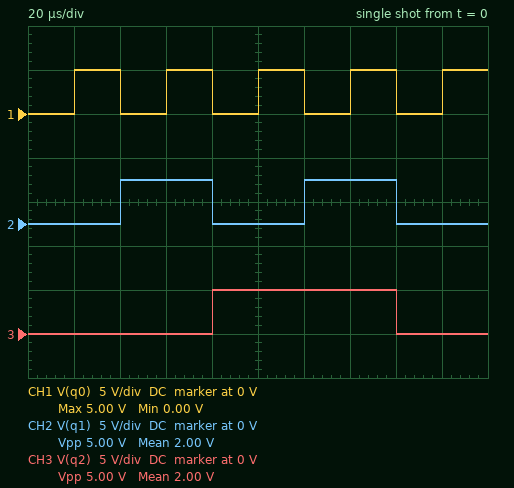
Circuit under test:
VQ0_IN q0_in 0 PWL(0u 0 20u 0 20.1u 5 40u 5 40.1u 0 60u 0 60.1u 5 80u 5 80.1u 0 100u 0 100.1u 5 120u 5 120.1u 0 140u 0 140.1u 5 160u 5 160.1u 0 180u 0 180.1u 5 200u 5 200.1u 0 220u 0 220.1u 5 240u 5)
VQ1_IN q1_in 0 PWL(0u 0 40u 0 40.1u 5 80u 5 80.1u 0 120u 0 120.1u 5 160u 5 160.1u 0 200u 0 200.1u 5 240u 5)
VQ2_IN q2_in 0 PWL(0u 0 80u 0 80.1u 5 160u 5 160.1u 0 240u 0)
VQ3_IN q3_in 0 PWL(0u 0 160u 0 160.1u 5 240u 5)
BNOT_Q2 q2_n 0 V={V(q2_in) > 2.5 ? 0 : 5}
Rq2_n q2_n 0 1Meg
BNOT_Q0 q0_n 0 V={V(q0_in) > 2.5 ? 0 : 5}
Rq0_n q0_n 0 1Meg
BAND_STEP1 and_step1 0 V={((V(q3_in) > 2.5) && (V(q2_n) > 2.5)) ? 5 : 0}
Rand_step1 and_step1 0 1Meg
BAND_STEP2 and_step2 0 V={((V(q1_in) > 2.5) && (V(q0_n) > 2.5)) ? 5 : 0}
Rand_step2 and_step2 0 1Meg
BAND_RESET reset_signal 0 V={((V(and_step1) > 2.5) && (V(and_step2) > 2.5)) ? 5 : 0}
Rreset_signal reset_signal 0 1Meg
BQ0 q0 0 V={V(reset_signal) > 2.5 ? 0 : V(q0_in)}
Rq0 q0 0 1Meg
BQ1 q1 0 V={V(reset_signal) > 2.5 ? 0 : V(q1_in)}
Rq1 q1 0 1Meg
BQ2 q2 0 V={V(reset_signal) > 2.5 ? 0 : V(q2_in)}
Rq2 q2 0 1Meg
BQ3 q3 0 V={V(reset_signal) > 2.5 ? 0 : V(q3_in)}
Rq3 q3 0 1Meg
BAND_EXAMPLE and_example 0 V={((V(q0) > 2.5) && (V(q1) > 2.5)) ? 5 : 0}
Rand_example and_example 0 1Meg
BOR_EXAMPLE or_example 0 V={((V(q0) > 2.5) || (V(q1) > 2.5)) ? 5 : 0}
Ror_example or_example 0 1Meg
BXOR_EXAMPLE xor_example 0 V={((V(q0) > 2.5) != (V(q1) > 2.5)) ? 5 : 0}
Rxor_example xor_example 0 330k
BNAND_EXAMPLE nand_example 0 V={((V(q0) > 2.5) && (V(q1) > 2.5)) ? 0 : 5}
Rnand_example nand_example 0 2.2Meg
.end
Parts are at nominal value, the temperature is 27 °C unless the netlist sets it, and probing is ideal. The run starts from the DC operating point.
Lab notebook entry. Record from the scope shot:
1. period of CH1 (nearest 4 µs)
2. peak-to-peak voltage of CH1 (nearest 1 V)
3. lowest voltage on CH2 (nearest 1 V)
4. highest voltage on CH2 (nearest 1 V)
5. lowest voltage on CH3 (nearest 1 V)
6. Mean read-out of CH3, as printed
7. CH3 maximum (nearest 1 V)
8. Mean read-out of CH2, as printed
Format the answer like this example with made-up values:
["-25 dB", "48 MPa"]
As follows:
["40 µs", "5 V", "0 V", "5 V", "0 V", "2.00 V", "5 V", "2.00 V"]
